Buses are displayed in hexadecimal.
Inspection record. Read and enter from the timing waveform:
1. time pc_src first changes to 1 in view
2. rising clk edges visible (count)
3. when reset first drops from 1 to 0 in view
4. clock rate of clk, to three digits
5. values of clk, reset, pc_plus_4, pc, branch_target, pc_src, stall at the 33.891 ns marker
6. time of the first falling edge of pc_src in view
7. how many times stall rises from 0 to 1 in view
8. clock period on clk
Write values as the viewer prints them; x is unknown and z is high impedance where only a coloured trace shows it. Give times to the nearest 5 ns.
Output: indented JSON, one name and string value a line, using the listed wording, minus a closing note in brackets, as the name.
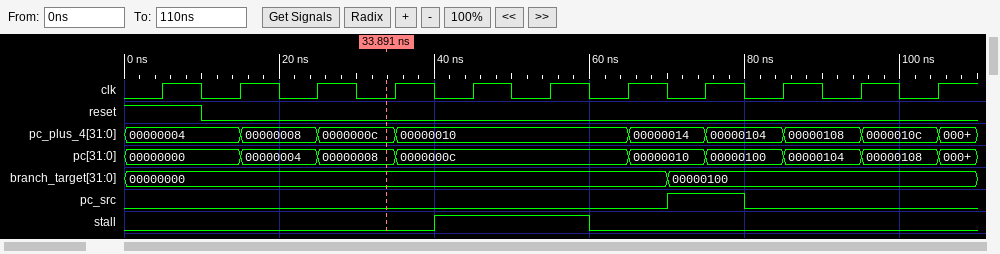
{
  "time pc_src first changes to 1 in view": "70 ns",
  "rising clk edges visible": "11",
  "when reset first drops from 1 to 0 in view": "10 ns",
  "clock rate of clk, to three digits": "100 MHz",
  "values of clk, reset, pc_plus_4, pc, branch_target, pc_src, stall at the 33.891 ns marker": "clk=0, reset=0, pc_plus_4=0000000c, pc=00000008, branch_target=00000000, pc_src=0, stall=0",
  "time of the first falling edge of pc_src in view": "80 ns",
  "how many times stall rises from 0 to 1 in view": "1",
  "clock period on clk": "10 ns"
}
